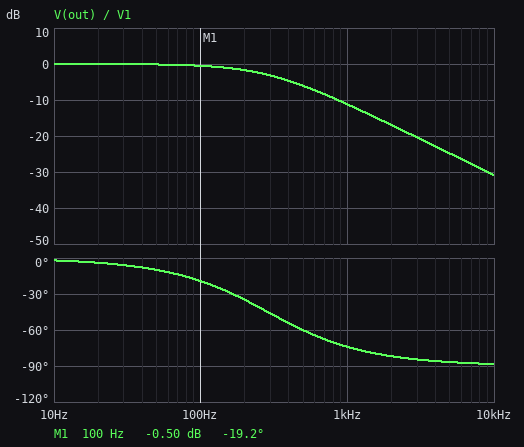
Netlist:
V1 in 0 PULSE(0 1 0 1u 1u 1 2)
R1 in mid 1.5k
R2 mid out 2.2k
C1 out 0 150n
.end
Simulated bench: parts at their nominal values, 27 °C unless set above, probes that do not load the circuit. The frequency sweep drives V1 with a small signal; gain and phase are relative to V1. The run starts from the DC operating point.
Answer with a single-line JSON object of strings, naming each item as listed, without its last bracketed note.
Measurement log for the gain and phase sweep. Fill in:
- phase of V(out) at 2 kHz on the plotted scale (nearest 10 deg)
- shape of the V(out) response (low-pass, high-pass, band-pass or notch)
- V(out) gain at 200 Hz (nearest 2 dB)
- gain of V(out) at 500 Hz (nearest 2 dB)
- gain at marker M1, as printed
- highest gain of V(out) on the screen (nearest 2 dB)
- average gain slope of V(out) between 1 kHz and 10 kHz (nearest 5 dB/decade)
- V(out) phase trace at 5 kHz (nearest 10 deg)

{"phase of V(out) at 2 kHz on the plotted scale": "-80 deg", "shape of the V(out) response": "low-pass", "V(out) gain at 200 Hz": "-2 dB", "gain of V(out) at 500 Hz": "-6 dB", "gain at marker M1, as printed": "-0.50 dB", "highest gain of V(out) on the screen": "0 dB", "average gain slope of V(out) between 1 kHz and 10 kHz": "-20 dB/decade", "V(out) phase trace at 5 kHz": "-90 deg"}
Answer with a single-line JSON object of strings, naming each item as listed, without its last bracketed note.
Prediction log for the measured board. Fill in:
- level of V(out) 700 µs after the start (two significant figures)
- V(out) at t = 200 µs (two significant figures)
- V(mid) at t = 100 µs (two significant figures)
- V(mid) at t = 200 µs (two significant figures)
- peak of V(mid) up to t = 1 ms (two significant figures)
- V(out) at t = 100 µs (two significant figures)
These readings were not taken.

{"level of V(out) 700 µs after the start": "720 mV", "V(out) at t = 200 µs": "300 mV", "V(mid) at t = 100 µs": "660 mV", "V(mid) at t = 200 µs": "720 mV", "peak of V(mid) up to t = 1 ms": "930 mV", "V(out) at t = 100 µs": "160 mV"}
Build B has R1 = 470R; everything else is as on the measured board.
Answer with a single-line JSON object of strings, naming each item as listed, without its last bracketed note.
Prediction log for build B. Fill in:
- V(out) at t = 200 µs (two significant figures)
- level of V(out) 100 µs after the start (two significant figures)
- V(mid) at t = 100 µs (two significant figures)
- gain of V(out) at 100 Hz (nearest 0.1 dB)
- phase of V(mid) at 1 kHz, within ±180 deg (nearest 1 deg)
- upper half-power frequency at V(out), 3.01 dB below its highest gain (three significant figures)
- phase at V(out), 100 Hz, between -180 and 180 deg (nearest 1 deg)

{"V(out) at t = 200 µs": "390 mV", "level of V(out) 100 µs after the start": "220 mV", "V(mid) at t = 100 µs": "860 mV", "gain of V(out) at 100 Hz": "-0.3 dB", "phase of V(mid) at 1 kHz, within ±180 deg": "-4 deg", "upper half-power frequency at V(out), 3.01 dB below its highest gain": "397 Hz", "phase at V(out), 100 Hz, between -180 and 180 deg": "-14 deg"}
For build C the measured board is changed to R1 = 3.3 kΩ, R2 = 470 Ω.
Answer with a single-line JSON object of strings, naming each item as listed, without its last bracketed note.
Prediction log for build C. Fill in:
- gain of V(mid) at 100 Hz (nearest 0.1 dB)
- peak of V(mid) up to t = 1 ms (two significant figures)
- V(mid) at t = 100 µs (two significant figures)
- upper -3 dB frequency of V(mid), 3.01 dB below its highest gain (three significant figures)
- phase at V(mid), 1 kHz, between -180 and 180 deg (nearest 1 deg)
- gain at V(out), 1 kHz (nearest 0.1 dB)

{"gain of V(mid) at 100 Hz": "-0.5 dB", "peak of V(mid) up to t = 1 ms": "850 mV", "V(mid) at t = 100 µs": "270 mV", "upper -3 dB frequency of V(mid), 3.01 dB below its highest gain": "286 Hz", "phase at V(mid), 1 kHz, between -180 and 180 deg": "-50 deg", "gain at V(out), 1 kHz": "-11.3 dB"}
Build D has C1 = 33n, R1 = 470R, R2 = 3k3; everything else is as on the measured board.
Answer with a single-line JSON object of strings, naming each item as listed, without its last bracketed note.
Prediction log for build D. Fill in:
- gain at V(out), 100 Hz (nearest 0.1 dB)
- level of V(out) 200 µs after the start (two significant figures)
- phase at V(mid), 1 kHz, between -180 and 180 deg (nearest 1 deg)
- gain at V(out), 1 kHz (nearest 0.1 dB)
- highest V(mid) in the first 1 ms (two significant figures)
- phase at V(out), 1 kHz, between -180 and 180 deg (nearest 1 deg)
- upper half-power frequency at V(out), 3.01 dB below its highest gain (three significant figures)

{"gain at V(out), 100 Hz": "0 dB", "level of V(out) 200 µs after the start": "800 mV", "phase at V(mid), 1 kHz, between -180 and 180 deg": "-4 deg", "gain at V(out), 1 kHz": "-2.1 dB", "highest V(mid) in the first 1 ms": "1.0 V", "phase at V(out), 1 kHz, between -180 and 180 deg": "-38 deg", "upper half-power frequency at V(out), 3.01 dB below its highest gain": "1.28 kHz"}
